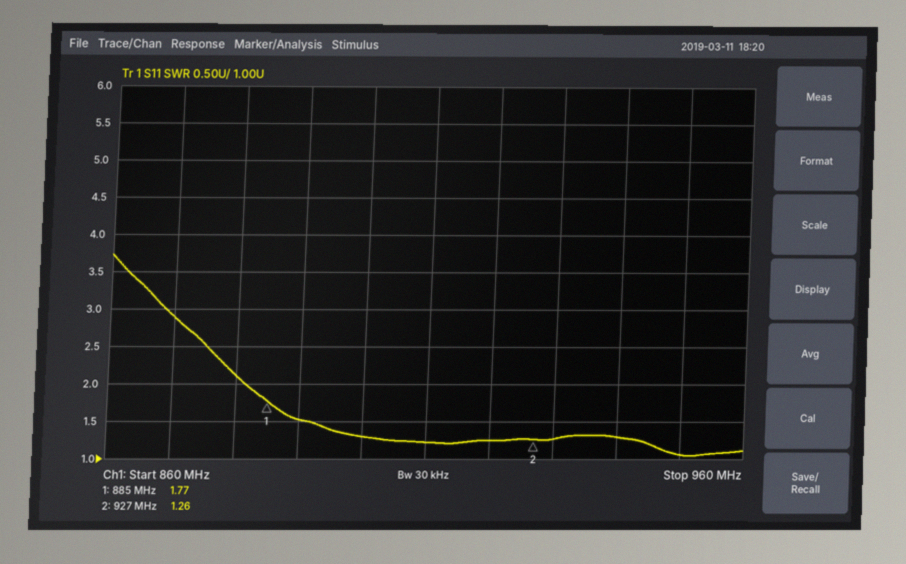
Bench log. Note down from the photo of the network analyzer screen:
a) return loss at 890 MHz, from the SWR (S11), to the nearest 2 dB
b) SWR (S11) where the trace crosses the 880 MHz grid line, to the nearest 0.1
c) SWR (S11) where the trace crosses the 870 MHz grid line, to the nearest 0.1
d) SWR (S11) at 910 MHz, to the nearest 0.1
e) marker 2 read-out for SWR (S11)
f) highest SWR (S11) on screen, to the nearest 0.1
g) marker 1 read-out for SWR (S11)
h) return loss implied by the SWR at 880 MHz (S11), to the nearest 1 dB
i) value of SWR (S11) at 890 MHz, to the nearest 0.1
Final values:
14 dB
2.1
2.9
1.2
1.26
3.7
1.77
9 dB
1.5
